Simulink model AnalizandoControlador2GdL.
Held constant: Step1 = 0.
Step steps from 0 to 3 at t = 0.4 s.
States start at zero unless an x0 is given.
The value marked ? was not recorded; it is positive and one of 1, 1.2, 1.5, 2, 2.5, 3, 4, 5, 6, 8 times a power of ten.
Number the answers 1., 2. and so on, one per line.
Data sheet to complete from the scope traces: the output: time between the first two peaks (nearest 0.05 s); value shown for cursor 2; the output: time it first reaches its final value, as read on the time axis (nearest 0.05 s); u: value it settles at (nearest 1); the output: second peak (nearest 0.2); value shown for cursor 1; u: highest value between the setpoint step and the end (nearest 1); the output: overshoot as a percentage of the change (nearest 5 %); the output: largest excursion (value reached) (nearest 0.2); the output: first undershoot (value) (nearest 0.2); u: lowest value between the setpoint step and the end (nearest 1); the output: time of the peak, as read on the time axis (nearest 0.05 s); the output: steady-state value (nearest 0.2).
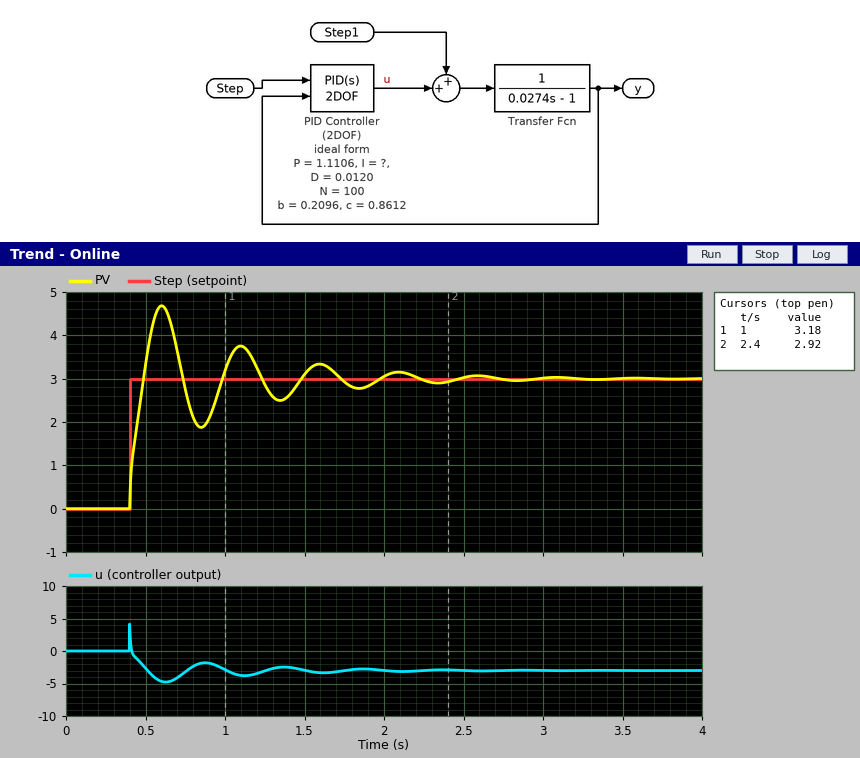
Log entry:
1. 0.50 s
2. 2.92
3. 0.50 s
4. -3
5. 3.8
6. 3.18
7. 4
8. 55 %
9. 4.6
10. 1.8
11. -5
12. 0.60 s
13. 3.0
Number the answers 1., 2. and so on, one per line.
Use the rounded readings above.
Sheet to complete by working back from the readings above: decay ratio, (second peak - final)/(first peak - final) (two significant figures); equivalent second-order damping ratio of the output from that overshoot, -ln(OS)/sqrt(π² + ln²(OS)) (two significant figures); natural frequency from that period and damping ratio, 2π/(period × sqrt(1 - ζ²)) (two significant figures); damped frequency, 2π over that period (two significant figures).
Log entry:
1. 0.50
2. 0.19
3. 13 rad/s
4. 13 rad/s
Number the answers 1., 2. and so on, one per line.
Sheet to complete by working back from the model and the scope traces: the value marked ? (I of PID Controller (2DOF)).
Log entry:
1. 6
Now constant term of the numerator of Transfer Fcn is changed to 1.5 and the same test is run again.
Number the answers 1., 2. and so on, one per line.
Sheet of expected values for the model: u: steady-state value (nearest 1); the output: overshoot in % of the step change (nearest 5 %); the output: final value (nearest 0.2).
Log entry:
1. -2
2. 10 %
3. 3.0
